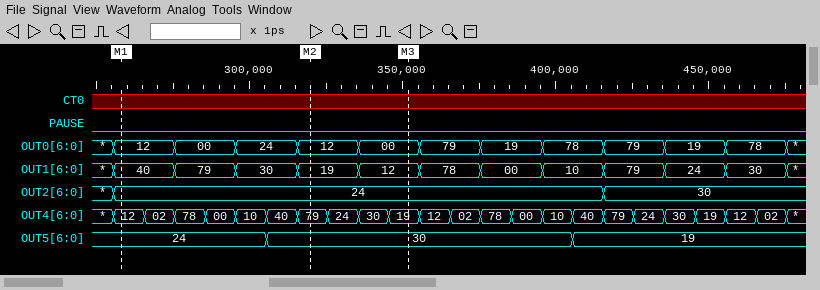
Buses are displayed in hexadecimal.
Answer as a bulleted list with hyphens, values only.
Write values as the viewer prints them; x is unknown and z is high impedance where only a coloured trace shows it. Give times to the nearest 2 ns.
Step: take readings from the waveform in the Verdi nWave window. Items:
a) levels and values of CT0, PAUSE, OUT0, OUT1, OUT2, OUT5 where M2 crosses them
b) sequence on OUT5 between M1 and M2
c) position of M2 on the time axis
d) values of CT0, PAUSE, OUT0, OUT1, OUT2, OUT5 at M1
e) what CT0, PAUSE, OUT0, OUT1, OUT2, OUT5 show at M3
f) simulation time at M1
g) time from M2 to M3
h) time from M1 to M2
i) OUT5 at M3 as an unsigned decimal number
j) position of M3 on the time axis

- CT0=x, PAUSE=0, OUT0=12, OUT1=19, OUT2=24, OUT5=30
- 24, 30
- 320 ns
- CT0=x, PAUSE=0, OUT0=12, OUT1=40, OUT2=24, OUT5=24
- CT0=x, PAUSE=0, OUT0=00, OUT1=12, OUT2=24, OUT5=30
- 258 ns
- 32 ns
- 62 ns
- 48
- 352 ns
